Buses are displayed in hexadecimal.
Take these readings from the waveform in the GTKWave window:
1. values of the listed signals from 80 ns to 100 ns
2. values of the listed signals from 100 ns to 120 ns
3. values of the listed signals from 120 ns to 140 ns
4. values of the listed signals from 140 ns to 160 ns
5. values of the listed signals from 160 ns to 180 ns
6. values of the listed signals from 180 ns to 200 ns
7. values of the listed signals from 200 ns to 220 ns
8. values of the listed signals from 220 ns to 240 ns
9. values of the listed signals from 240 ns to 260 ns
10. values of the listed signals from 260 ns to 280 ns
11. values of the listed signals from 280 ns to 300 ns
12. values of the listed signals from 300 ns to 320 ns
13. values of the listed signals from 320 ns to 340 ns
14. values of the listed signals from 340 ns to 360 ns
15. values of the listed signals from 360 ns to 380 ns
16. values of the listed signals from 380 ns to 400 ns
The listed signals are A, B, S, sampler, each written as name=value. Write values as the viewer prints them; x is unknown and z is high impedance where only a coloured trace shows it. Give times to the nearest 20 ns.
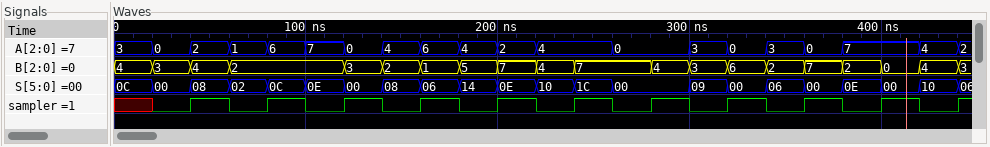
A=6, B=2, S=0C, sampler=1
A=7, B=2, S=0E, sampler=0
A=0, B=3, S=00, sampler=1
A=4, B=2, S=08, sampler=0
A=6, B=1, S=06, sampler=1
A=4, B=5, S=14, sampler=0
A=2, B=7, S=0E, sampler=1
A=4, B=4, S=10, sampler=0
A=4, B=7, S=1C, sampler=1
A=0, B=7, S=00, sampler=0
A=0, B=4, S=00, sampler=1
A=3, B=3, S=09, sampler=0
A=0, B=6, S=00, sampler=1
A=3, B=2, S=06, sampler=0
A=0, B=7, S=00, sampler=1
A=7, B=2, S=0E, sampler=0
